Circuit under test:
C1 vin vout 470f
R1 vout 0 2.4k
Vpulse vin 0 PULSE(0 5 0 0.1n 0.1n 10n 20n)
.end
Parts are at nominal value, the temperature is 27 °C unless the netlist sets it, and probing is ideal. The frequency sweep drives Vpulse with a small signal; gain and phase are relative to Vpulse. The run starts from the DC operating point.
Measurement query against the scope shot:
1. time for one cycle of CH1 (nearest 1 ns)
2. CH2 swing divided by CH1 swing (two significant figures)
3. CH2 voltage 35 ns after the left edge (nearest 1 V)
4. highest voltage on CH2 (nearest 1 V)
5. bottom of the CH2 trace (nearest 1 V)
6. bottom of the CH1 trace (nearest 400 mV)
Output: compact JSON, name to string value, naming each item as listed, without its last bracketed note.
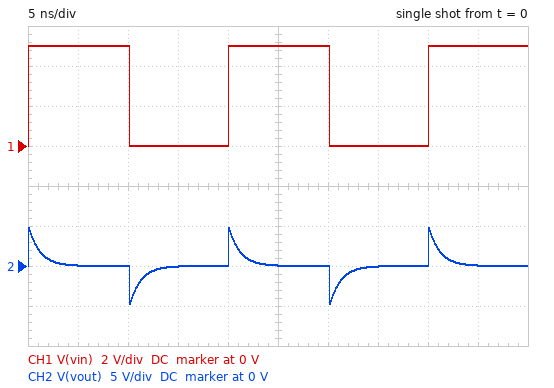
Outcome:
{"time for one cycle of CH1": "20 ns", "CH2 swing divided by CH1 swing": "1.9", "CH2 voltage 35 ns after the left edge": "0 V", "highest voltage on CH2": "5 V", "bottom of the CH2 trace": "-5 V", "bottom of the CH1 trace": "0 V"}
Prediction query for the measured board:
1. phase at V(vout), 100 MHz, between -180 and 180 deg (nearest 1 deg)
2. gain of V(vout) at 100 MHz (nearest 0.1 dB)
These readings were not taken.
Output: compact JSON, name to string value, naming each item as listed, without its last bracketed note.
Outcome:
{"phase at V(vout), 100 MHz, between -180 and 180 deg": "55 deg", "gain of V(vout) at 100 MHz": "-4.8 dB"}
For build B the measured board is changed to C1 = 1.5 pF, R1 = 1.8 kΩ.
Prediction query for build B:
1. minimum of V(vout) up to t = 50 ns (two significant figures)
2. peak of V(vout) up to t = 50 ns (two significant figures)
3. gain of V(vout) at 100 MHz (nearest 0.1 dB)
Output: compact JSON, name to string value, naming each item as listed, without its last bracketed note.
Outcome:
{"minimum of V(vout) up to t = 50 ns": "-4.8 V", "peak of V(vout) up to t = 50 ns": "4.9 V", "gain of V(vout) at 100 MHz": "-1.3 dB"}
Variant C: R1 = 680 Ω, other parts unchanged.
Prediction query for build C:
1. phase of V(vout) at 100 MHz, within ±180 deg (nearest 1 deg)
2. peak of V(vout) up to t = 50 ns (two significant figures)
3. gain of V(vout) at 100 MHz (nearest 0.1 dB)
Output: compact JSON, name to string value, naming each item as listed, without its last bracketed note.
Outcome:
{"phase of V(vout) at 100 MHz, within ±180 deg": "79 deg", "peak of V(vout) up to t = 50 ns": "4.3 V", "gain of V(vout) at 100 MHz": "-14.1 dB"}
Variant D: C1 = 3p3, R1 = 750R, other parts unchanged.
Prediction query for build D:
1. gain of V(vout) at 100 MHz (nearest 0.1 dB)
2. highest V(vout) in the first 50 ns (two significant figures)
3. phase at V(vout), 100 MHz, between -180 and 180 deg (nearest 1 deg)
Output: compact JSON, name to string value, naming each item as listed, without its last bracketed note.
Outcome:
{"gain of V(vout) at 100 MHz": "-1.5 dB", "highest V(vout) in the first 50 ns": "4.9 V", "phase at V(vout), 100 MHz, between -180 and 180 deg": "33 deg"}
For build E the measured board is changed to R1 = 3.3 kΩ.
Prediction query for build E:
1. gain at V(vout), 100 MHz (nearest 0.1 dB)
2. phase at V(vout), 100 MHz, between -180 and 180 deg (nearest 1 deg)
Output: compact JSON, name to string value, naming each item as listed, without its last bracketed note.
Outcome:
{"gain at V(vout), 100 MHz": "-3.1 dB", "phase at V(vout), 100 MHz, between -180 and 180 deg": "46 deg"}
